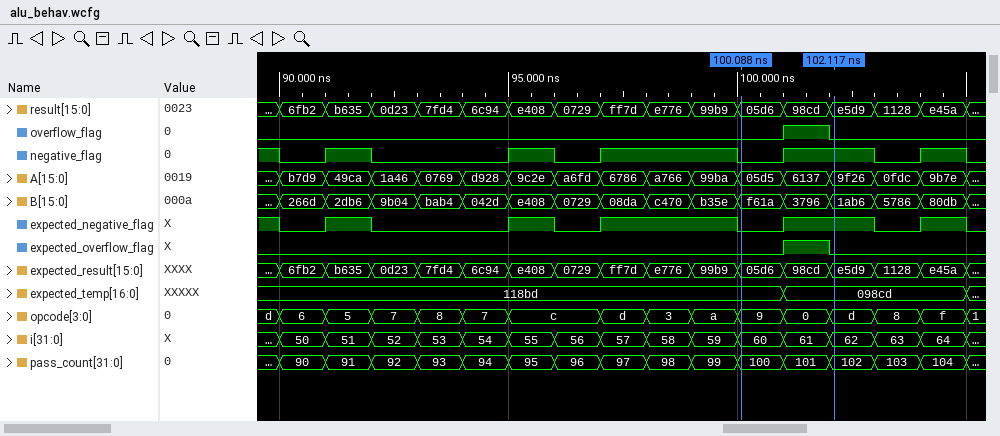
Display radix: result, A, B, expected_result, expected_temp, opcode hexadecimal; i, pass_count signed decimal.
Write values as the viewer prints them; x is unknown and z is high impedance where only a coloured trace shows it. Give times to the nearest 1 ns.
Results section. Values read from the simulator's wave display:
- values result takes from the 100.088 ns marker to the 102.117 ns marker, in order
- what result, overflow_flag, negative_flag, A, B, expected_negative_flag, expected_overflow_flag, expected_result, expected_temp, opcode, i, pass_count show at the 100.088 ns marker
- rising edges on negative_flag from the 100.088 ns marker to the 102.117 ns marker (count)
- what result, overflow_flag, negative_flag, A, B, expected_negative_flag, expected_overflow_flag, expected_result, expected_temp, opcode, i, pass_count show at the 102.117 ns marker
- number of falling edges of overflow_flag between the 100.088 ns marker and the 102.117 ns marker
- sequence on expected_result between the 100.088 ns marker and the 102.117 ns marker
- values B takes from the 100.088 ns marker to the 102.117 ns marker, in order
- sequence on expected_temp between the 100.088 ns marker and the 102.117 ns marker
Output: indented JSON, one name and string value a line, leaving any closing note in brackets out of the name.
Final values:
{
  "values result takes from the 100.088 ns marker to the 102.117 ns marker, in order": "05d6, 98cd, e5d9",
  "what result, overflow_flag, negative_flag, A, B, expected_negative_flag, expected_overflow_flag, expected_result, expected_temp, opcode, i, pass_count show at the 100.088 ns marker": "result=05d6, overflow_flag=0, negative_flag=0, A=05d5, B=f61a, expected_negative_flag=0, expected_overflow_flag=0, expected_result=05d6, expected_temp=118bd, opcode=9, i=60, pass_count=100",
  "rising edges on negative_flag from the 100.088 ns marker to the 102.117 ns marker": "1",
  "what result, overflow_flag, negative_flag, A, B, expected_negative_flag, expected_overflow_flag, expected_result, expected_temp, opcode, i, pass_count show at the 102.117 ns marker": "result=e5d9, overflow_flag=0, negative_flag=1, A=9f26, B=1ab6, expected_negative_flag=1, expected_overflow_flag=0, expected_result=e5d9, expected_temp=098cd, opcode=d, i=62, pass_count=102",
  "number of falling edges of overflow_flag between the 100.088 ns marker and the 102.117 ns marker": "1",
  "sequence on expected_result between the 100.088 ns marker and the 102.117 ns marker": "05d6, 98cd, e5d9",
  "values B takes from the 100.088 ns marker to the 102.117 ns marker, in order": "f61a, 3796, 1ab6",
  "sequence on expected_temp between the 100.088 ns marker and the 102.117 ns marker": "118bd, 098cd"
}
